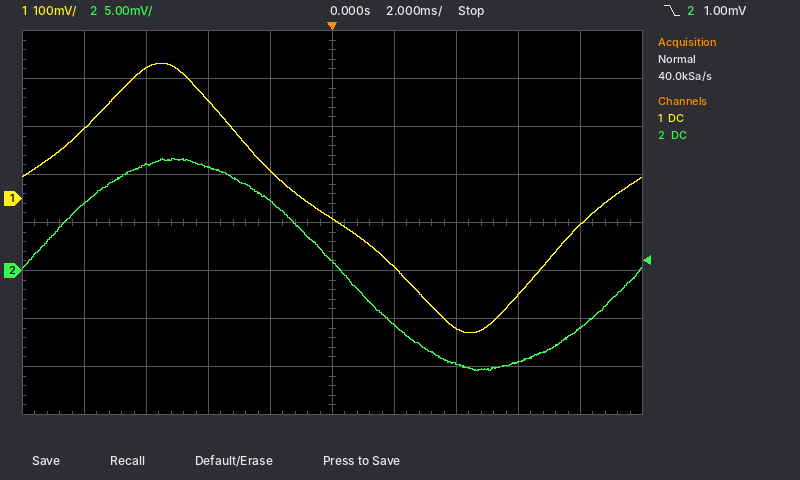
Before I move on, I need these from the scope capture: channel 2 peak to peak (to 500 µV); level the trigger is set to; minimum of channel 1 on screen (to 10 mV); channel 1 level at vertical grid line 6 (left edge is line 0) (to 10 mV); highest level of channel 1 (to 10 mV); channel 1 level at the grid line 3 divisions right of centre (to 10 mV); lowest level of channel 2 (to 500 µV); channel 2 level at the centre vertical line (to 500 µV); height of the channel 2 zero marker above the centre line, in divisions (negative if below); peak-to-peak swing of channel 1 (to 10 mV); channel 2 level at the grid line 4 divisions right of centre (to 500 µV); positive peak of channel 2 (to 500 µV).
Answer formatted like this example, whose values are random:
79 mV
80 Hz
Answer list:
22.0 mV
1.00 mV
-280 mV
-140 mV
280 mV
-200 mV
-10.5 mV
1.0 mV
-1.0 div
560 mV
-6.0 mV
11.5 mV
